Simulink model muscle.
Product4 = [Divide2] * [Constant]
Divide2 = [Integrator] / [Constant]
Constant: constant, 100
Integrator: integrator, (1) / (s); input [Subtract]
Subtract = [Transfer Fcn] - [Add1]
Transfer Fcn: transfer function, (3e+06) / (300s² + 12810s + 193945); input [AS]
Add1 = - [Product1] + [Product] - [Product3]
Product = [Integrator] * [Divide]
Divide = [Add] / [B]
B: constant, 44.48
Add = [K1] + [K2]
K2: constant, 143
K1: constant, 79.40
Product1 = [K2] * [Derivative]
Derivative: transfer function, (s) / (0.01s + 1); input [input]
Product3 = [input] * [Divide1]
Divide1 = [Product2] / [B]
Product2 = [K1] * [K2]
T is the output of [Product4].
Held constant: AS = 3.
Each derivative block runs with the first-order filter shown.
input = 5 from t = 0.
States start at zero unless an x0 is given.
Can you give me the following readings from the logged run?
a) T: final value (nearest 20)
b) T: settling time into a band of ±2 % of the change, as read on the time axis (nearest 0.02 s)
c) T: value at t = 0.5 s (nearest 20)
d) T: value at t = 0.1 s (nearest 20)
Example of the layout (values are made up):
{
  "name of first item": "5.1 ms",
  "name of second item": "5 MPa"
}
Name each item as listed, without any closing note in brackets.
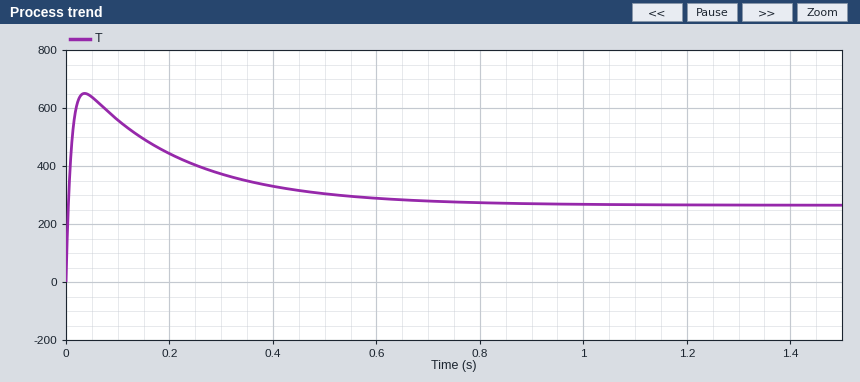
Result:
{
  "T: final value": "260",
  "T: settling time into a band of ±2 % of the change, as read on the time axis": "0.90 s",
  "T: value at t = 0.5 s": "300",
  "T: value at t = 0.1 s": "560"
}
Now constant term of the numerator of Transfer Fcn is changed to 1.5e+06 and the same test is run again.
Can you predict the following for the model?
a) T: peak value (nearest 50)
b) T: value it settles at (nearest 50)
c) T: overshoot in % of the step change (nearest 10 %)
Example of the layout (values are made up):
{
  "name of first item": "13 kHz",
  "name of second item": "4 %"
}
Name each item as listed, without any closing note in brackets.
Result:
{
  "T: peak value": "650",
  "T: value it settles at": "250",
  "T: overshoot in % of the step change": "150 %"
}
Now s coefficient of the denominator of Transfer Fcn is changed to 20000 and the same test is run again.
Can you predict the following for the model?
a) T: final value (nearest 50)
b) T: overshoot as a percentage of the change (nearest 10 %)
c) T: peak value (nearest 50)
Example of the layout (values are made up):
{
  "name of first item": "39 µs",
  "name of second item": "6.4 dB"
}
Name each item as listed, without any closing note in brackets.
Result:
{
  "T: final value": "250",
  "T: overshoot as a percentage of the change": "150 %",
  "T: peak value": "650"
}
